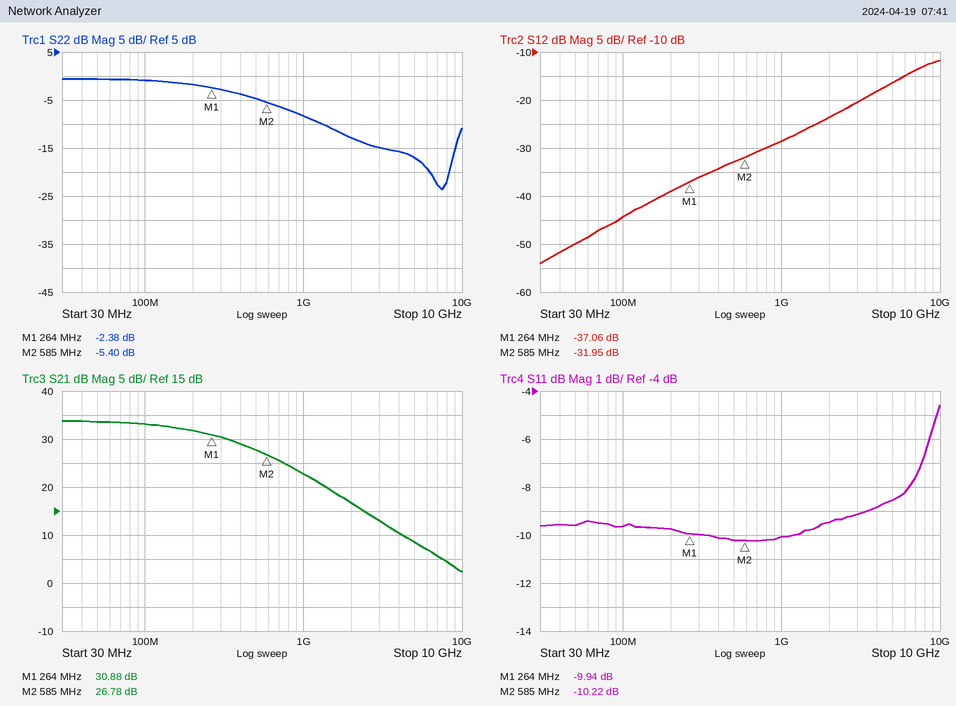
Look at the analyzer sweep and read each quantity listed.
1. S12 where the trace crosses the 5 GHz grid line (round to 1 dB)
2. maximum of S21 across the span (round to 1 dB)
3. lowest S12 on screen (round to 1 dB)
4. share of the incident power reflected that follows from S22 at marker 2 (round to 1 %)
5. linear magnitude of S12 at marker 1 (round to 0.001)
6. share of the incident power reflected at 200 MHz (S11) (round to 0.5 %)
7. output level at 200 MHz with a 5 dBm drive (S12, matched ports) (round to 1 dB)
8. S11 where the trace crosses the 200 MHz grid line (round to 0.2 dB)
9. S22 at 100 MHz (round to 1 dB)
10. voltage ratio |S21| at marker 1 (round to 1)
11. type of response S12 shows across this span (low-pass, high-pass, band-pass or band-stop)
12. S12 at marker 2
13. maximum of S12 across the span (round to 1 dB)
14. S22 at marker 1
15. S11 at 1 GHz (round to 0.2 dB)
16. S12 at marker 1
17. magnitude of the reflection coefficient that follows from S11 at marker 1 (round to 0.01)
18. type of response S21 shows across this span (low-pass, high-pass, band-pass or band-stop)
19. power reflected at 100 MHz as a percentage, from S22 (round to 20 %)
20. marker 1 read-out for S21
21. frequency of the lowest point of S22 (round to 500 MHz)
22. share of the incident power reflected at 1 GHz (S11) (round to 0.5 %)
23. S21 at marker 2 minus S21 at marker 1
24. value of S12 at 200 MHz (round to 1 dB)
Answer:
-16 dB
34 dB
-54 dB
29 %
0.014
10.5 %
-34 dBm
-9.8 dB
-1 dB
35
high-pass
-31.95 dB
-12 dB
-2.38 dB
-10.0 dB
-37.06 dB
0.32
low-pass
80 %
30.88 dB
7.5 GHz
10.0 %
-4.10 dB
-39 dB
